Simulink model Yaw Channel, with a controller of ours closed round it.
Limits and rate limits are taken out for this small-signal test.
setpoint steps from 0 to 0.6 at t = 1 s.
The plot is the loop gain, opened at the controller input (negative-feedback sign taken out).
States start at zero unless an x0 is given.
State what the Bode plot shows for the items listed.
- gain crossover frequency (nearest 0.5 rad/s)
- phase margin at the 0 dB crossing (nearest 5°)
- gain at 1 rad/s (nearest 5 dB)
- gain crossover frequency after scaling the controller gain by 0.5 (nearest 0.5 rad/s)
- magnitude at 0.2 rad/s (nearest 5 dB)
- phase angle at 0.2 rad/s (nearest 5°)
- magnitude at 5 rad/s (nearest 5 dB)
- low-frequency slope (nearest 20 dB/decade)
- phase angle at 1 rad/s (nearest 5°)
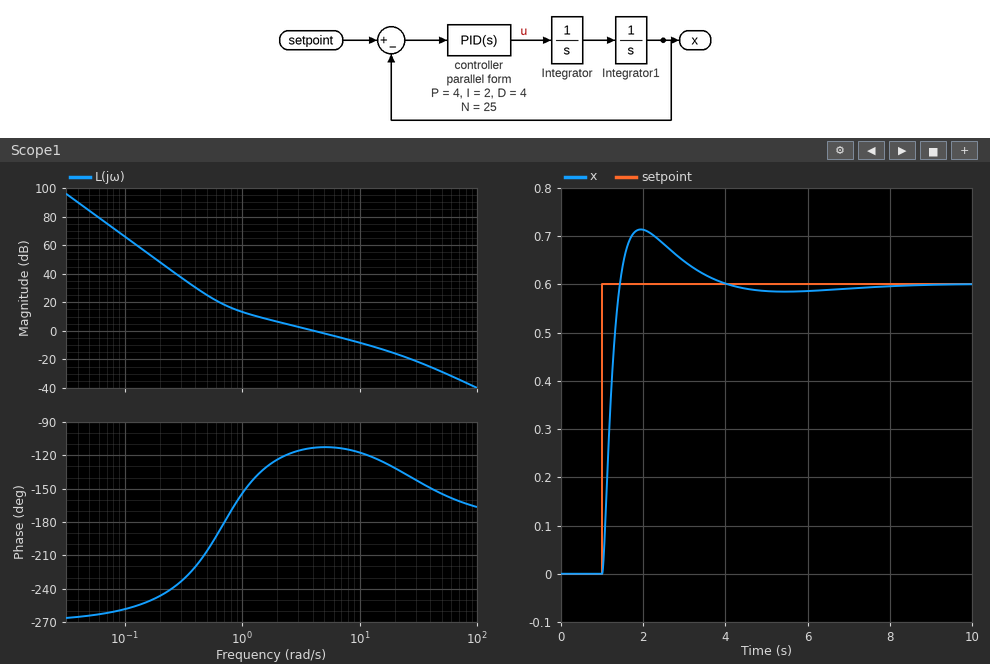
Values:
4.0 rad/s
65°
15 dB
2.0 rad/s
50 dB
-245°
0 dB
-60 dB/decade
-155°
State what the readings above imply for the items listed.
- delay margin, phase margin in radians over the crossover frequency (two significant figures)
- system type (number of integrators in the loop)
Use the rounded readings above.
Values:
0.28 s
3
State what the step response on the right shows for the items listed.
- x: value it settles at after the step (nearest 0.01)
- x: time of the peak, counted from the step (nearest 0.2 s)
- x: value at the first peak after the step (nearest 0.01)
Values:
0.60
1.0 s
0.71
